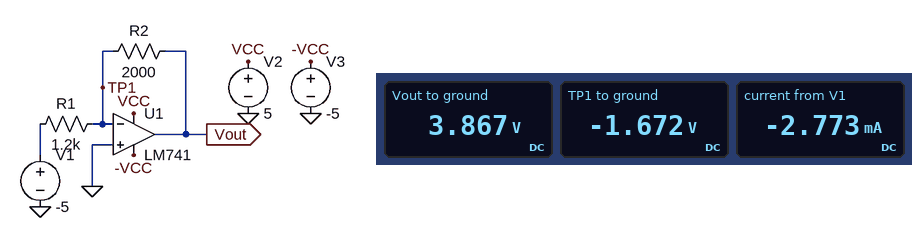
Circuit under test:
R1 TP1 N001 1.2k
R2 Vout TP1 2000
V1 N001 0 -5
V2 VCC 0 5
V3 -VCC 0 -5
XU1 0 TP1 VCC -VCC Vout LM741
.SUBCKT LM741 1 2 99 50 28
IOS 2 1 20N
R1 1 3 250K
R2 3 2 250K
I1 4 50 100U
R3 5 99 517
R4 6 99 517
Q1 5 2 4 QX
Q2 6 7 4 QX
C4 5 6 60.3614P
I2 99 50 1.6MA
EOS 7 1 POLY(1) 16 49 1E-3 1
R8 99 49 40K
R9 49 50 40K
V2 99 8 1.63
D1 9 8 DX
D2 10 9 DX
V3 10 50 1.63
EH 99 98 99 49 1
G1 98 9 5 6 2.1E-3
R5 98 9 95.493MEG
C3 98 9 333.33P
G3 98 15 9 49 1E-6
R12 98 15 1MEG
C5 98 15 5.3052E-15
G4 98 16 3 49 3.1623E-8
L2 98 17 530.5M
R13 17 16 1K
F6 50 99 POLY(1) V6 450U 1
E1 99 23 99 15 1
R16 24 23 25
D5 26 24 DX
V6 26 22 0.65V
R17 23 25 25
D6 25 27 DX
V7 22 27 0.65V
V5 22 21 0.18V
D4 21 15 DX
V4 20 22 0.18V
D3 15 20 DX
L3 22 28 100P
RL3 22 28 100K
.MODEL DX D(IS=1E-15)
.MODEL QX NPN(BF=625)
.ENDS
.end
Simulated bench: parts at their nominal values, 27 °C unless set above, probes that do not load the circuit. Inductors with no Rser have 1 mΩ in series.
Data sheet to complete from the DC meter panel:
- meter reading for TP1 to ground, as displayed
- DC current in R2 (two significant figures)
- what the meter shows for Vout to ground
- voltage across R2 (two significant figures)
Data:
-1.672 V
2.8 mA
3.867 V
5.5 V
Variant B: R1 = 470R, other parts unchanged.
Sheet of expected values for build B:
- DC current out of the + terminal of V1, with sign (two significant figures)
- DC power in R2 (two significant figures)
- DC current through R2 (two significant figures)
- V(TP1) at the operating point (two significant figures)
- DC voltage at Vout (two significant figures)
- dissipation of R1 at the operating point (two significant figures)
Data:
-3.6 mA
26 mW
3.6 mA
-3.3 V
3.8 V
6.0 mW
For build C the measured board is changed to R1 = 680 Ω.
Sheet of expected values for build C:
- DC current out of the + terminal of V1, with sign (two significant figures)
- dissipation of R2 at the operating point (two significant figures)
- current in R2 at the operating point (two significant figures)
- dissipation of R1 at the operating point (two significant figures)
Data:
-3.3 mA
22 mW
3.3 mA
7.4 mW
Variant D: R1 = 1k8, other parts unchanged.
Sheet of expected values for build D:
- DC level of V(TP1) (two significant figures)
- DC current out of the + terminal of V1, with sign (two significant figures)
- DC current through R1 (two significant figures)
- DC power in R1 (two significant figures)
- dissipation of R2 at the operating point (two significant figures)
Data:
-790 mV
-2.3 mA
2.3 mA
9.8 mW
11 mW
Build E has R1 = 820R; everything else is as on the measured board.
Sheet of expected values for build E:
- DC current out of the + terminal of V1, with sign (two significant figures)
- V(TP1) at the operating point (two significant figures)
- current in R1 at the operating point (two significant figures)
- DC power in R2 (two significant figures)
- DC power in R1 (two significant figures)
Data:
-3.1 mA
-2.4 V
3.1 mA
20 mW
8.1 mW
